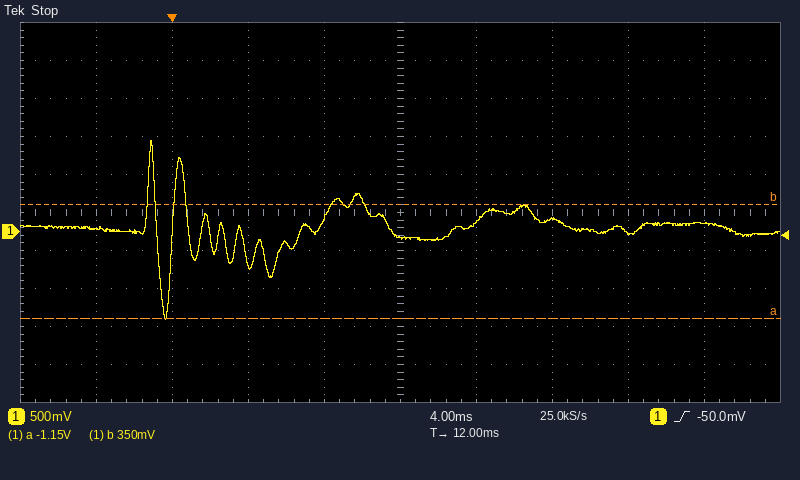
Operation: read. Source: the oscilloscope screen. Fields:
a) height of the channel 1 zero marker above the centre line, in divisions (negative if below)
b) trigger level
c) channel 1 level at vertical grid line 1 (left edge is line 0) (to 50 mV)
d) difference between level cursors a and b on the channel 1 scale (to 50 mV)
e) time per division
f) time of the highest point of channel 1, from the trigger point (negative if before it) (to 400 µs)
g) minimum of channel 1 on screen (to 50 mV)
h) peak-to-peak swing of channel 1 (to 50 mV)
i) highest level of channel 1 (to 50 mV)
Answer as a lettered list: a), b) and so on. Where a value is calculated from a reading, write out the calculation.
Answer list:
a) -0.5 div
b) -50.0 mV
c) 50 mV
d) 1.50 V
e) 4 ms
f) -1.2 ms
g) -1.15 V
h) 1.20 V − (-1.15 V) = 2.35 V
i) 1.20 V
